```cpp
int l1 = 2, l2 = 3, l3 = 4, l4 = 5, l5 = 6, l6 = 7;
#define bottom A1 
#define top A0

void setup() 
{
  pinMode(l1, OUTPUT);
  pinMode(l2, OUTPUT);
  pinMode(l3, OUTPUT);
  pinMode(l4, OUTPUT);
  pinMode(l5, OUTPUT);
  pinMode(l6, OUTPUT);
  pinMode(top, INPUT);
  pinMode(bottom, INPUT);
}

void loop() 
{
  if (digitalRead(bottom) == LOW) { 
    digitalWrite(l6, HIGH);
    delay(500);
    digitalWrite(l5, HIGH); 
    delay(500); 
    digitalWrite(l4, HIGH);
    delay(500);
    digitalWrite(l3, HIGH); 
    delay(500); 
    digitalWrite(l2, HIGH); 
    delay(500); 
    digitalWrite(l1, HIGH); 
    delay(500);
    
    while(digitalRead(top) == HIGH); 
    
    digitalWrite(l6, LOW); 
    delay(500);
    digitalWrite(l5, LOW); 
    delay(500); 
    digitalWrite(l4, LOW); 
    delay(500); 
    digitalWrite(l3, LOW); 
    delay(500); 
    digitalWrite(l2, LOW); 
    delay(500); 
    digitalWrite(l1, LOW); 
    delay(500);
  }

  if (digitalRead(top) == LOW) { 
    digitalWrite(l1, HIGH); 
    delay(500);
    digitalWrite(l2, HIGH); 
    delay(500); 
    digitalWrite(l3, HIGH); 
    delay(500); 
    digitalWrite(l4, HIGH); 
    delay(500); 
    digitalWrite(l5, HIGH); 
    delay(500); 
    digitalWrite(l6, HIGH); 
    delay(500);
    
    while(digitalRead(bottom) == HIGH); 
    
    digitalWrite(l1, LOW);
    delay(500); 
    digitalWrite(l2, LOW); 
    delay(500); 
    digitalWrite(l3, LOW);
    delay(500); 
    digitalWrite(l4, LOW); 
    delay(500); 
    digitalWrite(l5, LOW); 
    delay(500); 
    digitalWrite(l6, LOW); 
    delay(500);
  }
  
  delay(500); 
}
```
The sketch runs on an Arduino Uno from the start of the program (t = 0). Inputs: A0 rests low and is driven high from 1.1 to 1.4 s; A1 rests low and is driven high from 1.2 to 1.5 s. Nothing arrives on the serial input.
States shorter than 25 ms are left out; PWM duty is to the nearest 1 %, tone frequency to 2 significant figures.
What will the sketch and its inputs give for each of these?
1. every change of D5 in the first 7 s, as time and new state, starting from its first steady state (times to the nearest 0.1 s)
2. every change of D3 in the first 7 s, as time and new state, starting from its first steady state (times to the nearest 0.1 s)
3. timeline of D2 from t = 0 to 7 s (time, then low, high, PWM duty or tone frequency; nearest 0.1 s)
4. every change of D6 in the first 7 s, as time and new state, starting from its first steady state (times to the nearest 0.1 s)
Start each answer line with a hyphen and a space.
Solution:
- 0 s low; 1 s high; 4 s low
- 0 s low; 2 s high; 5 s low; 6.5 s high
- 0 s low; 2.5 s high; 5.5 s low; 6 s high
- 0 s low; 0.5 s high; 3.5 s low
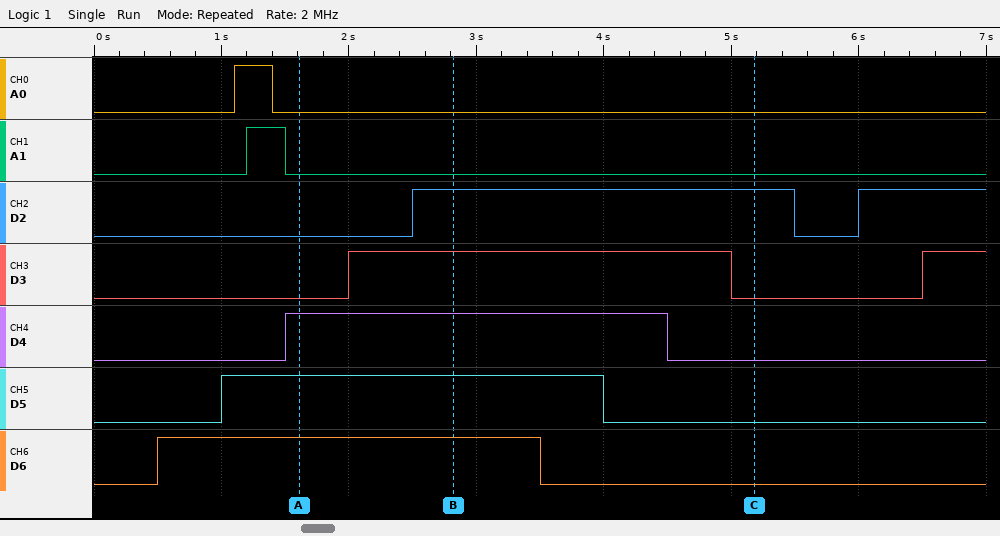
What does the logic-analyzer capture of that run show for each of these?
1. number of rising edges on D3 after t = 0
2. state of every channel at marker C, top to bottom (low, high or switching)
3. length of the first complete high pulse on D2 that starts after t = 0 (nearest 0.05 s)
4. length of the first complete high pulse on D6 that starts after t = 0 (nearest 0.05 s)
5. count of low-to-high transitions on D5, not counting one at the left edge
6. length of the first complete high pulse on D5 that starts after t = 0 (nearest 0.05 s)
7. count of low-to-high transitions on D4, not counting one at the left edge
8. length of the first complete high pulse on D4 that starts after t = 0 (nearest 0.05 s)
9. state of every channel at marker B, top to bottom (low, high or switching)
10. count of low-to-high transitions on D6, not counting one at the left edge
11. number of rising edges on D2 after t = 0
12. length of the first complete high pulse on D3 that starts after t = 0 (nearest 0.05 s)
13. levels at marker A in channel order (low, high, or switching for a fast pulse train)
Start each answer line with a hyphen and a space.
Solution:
- 2
- A0 low, A1 low, D2 high, D3 low, D4 low, D5 low, D6 low
- 3.00 s
- 3.00 s
- 1
- 3.00 s
- 1
- 3.00 s
- A0 low, A1 low, D2 high, D3 high, D4 high, D5 high, D6 high
- 1
- 2
- 3.00 s
- A0 low, A1 low, D2 low, D3 low, D4 high, D5 high, D6 high
